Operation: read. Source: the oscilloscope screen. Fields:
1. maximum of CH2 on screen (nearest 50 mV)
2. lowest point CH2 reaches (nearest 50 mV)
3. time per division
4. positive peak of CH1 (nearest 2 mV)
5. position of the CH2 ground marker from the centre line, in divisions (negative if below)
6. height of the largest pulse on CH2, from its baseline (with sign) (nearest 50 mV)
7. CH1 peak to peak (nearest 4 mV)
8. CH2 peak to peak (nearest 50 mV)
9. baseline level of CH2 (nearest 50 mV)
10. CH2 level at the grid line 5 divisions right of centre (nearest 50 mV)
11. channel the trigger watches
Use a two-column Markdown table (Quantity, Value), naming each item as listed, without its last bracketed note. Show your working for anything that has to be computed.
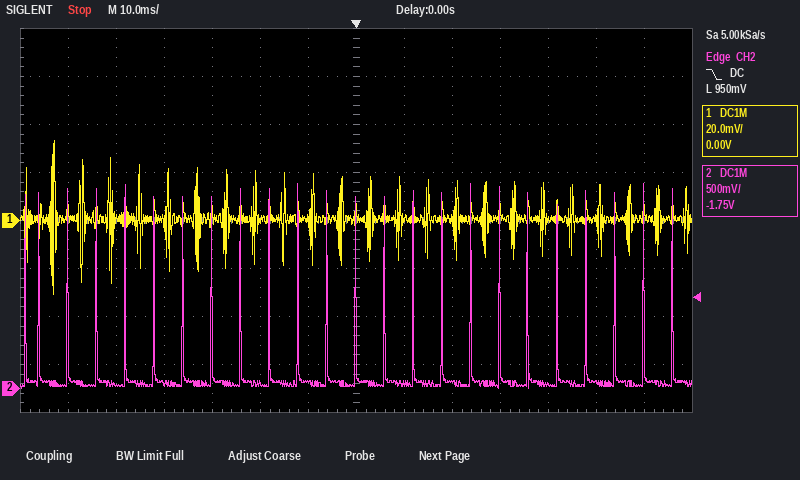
| Quantity | Value |
|---|---|
| maximum of CH2 on screen | 2.15 V |
| lowest point CH2 reaches | 0 mV |
| time per division | 10 ms |
| positive peak of CH1 | 34 mV |
| position of the CH2 ground marker from the centre line, in divisions | -3.5 div |
| height of the largest pulse on CH2, from its baseline (with sign) | 2.15 V − (50 mV) = +2.10 V |
| CH1 peak to peak | 64 mV |
| CH2 peak to peak | 2.15 V − (0 mV) = 2.15 V |
| baseline level of CH2 | 50 mV |
| CH2 level at the grid line 5 divisions right of centre | 50 mV |
| channel the trigger watches | CH2 |
